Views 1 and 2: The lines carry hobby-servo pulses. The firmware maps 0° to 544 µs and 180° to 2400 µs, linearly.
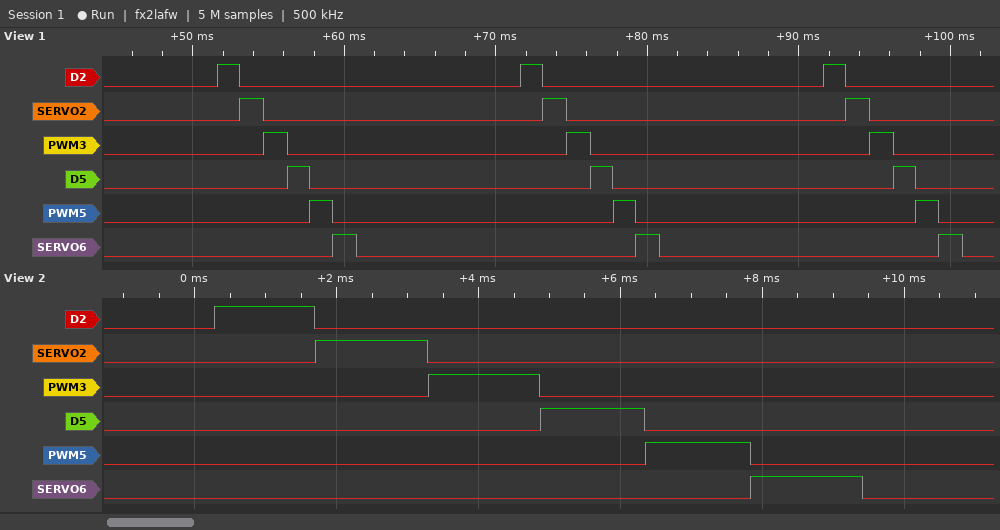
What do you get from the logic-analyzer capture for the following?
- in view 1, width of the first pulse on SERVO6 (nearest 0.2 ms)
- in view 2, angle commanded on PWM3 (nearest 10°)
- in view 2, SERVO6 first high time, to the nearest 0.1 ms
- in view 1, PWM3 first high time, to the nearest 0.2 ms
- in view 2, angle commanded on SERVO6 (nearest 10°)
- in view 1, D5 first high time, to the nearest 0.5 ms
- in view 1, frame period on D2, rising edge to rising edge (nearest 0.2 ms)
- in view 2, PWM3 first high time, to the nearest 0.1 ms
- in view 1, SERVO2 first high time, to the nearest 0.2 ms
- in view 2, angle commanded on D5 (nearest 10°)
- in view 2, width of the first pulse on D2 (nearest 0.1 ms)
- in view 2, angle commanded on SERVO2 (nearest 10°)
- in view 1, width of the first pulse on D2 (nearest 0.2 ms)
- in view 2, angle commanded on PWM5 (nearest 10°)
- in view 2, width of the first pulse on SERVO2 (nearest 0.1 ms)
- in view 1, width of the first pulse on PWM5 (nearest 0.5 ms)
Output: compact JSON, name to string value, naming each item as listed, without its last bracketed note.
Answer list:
{"in view 1, width of the first pulse on SERVO6": "1.6 ms", "in view 2, angle commanded on PWM3": "100°", "in view 2, SERVO6 first high time, to the nearest 0.1 ms": "1.6 ms", "in view 1, PWM3 first high time, to the nearest 0.2 ms": "1.6 ms", "in view 2, angle commanded on SERVO6": "100°", "in view 1, D5 first high time, to the nearest 0.5 ms": "1.5 ms", "in view 1, frame period on D2, rising edge to rising edge": "20.0 ms", "in view 2, PWM3 first high time, to the nearest 0.1 ms": "1.6 ms", "in view 1, SERVO2 first high time, to the nearest 0.2 ms": "1.6 ms", "in view 2, angle commanded on D5": "90°", "in view 2, width of the first pulse on D2": "1.4 ms", "in view 2, angle commanded on SERVO2": "100°", "in view 1, width of the first pulse on D2": "1.4 ms", "in view 2, angle commanded on PWM5": "90°", "in view 2, width of the first pulse on SERVO2": "1.6 ms", "in view 1, width of the first pulse on PWM5": "1.5 ms"}
